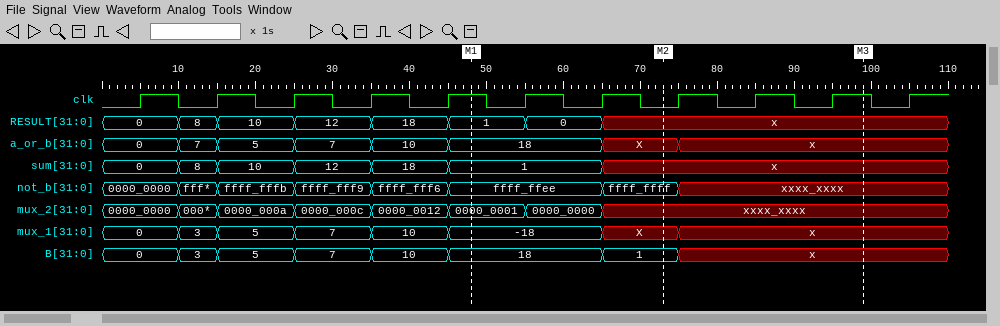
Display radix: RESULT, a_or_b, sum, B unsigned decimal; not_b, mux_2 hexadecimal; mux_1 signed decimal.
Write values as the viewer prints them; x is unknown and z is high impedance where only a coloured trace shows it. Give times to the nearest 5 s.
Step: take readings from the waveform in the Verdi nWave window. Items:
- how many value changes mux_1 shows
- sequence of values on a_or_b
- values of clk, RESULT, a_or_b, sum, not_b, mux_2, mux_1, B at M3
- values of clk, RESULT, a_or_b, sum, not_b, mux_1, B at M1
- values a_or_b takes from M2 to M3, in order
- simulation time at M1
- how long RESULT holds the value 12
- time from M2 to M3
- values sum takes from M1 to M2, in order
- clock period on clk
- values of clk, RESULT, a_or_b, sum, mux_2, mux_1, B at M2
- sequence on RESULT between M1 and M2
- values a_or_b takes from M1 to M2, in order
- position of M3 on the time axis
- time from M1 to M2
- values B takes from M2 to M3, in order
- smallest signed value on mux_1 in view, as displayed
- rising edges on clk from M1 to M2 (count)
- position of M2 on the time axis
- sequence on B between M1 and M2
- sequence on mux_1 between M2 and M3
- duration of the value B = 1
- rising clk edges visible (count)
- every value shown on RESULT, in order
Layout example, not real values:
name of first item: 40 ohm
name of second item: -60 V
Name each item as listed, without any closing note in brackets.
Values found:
how many value changes mux_1 shows: 7
sequence of values on a_or_b: 0, 7, 5, 7, 10, 18, X, x
values of clk, RESULT, a_or_b, sum, not_b, mux_2, mux_1, B at M3: clk=1, RESULT=x, a_or_b=x, sum=x, not_b=xxxx_xxxx, mux_2=xxxx_xxxx, mux_1=x, B=x
values of clk, RESULT, a_or_b, sum, not_b, mux_1, B at M1: clk=1, RESULT=1, a_or_b=18, sum=1, not_b=ffff_ffee, mux_1=-18, B=18
values a_or_b takes from M2 to M3, in order: X, x
simulation time at M1: 50 s
how long RESULT holds the value 12: 10 s
time from M2 to M3: 25 s
values sum takes from M1 to M2, in order: 1, x
clock period on clk: 10 s
values of clk, RESULT, a_or_b, sum, mux_2, mux_1, B at M2: clk=0, RESULT=x, a_or_b=X, sum=x, mux_2=xxxx_xxxx, mux_1=X, B=1
sequence on RESULT between M1 and M2: 1, 0, x
values a_or_b takes from M1 to M2, in order: 18, X
position of M3 on the time axis: 100 s
time from M1 to M2: 25 s
values B takes from M2 to M3, in order: 1, x
smallest signed value on mux_1 in view, as displayed: -18
rising edges on clk from M1 to M2: 2
position of M2 on the time axis: 75 s
sequence on B between M1 and M2: 18, 1
sequence on mux_1 between M2 and M3: X, x
duration of the value B = 1: 10 s
rising clk edges visible: 11
every value shown on RESULT, in order: 0, 8, 10, 12, 18, 1, 0, x
